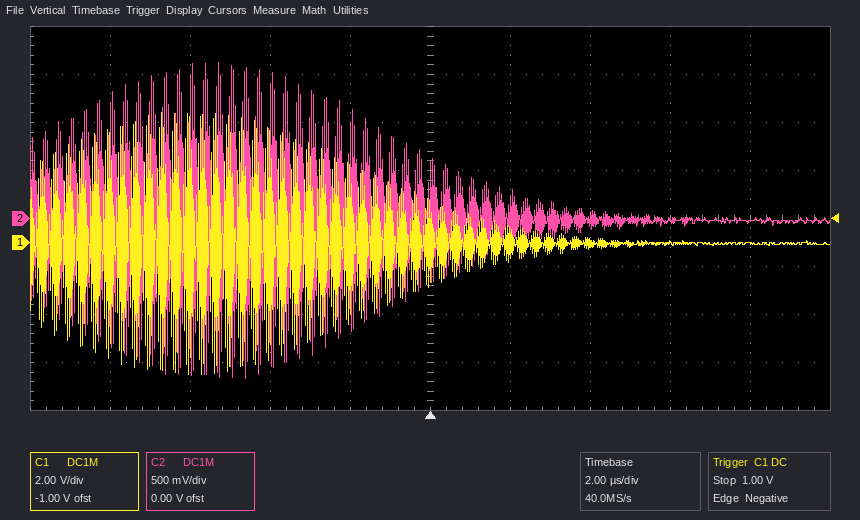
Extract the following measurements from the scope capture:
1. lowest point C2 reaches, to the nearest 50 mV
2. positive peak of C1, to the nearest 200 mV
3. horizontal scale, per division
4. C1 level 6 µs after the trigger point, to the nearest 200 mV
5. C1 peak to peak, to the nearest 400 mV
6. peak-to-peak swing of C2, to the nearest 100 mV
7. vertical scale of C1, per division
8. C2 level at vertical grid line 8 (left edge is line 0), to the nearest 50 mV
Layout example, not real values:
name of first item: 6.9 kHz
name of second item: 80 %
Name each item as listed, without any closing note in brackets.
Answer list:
lowest point C2 reaches, to the nearest 50 mV: -1.65 V
positive peak of C1, to the nearest 200 mV: 5.4 V
horizontal scale, per division: 2 µs
C1 level 6 µs after the trigger point, to the nearest 200 mV: 0.0 V
C1 peak to peak, to the nearest 400 mV: 10.8 V
peak-to-peak swing of C2, to the nearest 100 mV: 3.30 V
vertical scale of C1, per division: 2 V
C2 level at vertical grid line 8 (left edge is line 0), to the nearest 50 mV: 0 mV
